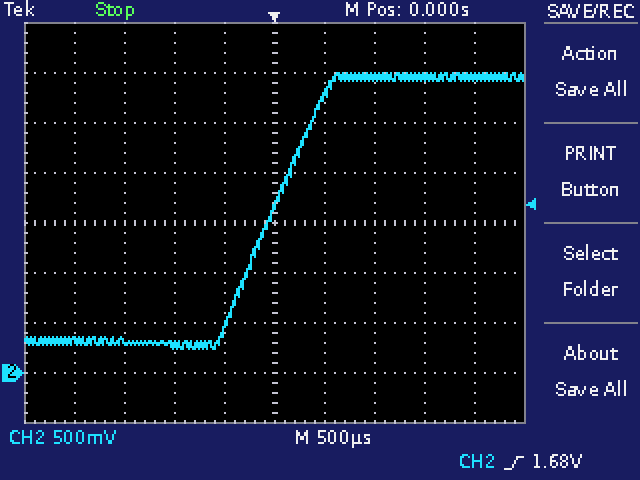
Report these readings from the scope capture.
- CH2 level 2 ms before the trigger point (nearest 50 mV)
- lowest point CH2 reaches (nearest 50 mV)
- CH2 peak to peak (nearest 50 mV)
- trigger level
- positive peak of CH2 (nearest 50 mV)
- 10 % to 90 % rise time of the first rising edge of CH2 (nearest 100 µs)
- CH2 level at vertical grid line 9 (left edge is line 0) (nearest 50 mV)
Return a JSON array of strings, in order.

["300 mV", "250 mV", "2.75 V", "1.68 V", "3.00 V", "900 µs", "2.95 V"]
